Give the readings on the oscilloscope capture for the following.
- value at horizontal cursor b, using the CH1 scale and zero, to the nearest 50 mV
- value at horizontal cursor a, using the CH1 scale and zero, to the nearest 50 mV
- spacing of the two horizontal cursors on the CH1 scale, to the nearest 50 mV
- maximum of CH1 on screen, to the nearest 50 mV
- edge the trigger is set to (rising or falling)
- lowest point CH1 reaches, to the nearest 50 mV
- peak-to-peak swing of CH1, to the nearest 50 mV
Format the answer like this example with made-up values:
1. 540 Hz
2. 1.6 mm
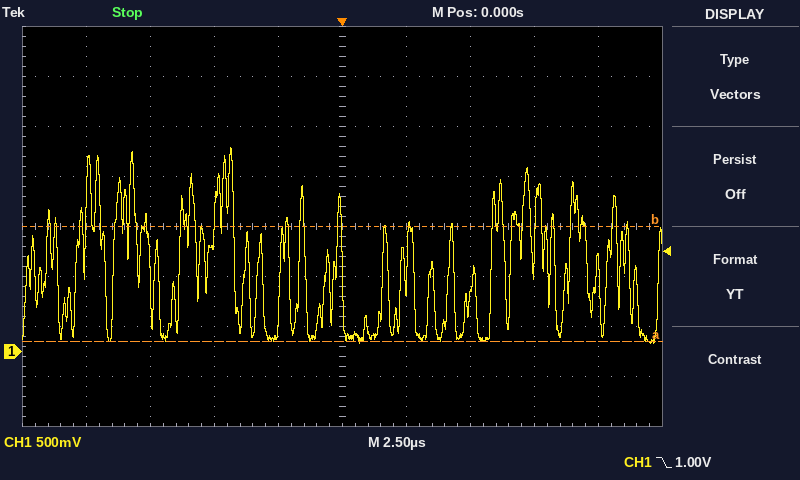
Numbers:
1. 1.25 V
2. 100 mV
3. 1.15 V
4. 2.05 V
5. falling
6. 100 mV
7. 1.95 V
